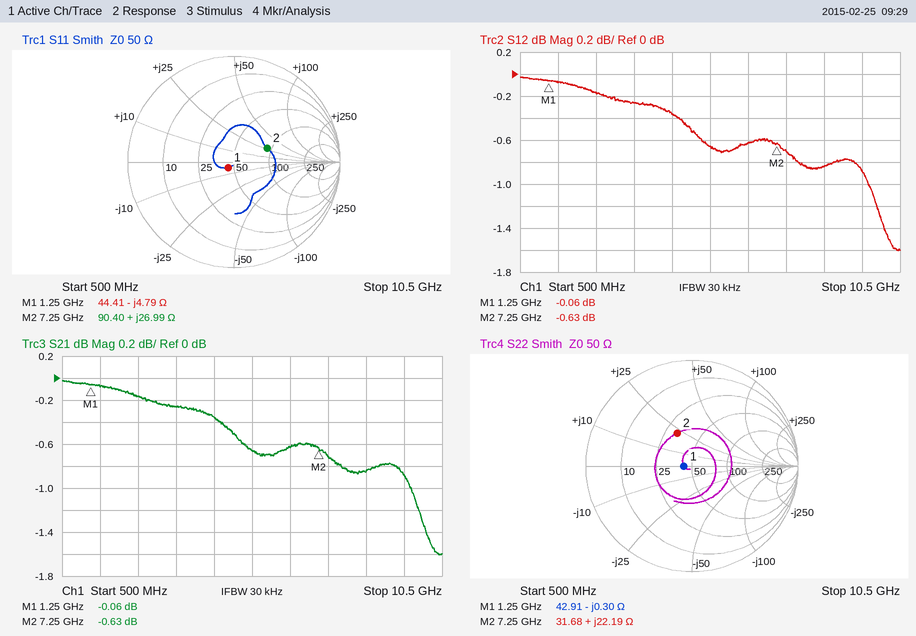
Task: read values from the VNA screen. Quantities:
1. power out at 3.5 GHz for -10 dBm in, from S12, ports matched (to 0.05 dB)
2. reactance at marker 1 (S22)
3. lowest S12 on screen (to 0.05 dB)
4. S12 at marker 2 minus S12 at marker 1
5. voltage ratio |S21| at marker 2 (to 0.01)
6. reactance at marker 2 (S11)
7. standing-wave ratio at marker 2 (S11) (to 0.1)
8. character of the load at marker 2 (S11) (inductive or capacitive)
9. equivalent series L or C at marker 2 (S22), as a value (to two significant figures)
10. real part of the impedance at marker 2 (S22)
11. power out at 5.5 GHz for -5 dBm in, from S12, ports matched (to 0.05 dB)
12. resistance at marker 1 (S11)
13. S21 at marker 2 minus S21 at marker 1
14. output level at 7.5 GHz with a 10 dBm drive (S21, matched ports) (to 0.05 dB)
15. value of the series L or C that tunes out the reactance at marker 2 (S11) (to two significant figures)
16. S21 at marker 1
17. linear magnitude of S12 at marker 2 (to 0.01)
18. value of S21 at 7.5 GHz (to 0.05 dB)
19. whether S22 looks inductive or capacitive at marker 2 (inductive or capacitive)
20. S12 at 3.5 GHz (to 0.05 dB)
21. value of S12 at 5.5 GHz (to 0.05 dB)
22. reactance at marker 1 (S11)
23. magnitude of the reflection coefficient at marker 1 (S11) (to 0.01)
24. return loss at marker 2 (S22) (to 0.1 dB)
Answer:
-10.25 dBm
-0.30 Ω
-1.60 dB
-0.57 dB
0.93
+26.99 Ω
2.0
inductive
490 pH
31.68 Ω
-5.65 dBm
44.41 Ω
-0.57 dB
9.30 dBm
810 fF
-0.06 dB
0.93
-0.70 dB
inductive
-0.25 dB
-0.65 dB
-4.79 Ω
0.08
9.4 dB
